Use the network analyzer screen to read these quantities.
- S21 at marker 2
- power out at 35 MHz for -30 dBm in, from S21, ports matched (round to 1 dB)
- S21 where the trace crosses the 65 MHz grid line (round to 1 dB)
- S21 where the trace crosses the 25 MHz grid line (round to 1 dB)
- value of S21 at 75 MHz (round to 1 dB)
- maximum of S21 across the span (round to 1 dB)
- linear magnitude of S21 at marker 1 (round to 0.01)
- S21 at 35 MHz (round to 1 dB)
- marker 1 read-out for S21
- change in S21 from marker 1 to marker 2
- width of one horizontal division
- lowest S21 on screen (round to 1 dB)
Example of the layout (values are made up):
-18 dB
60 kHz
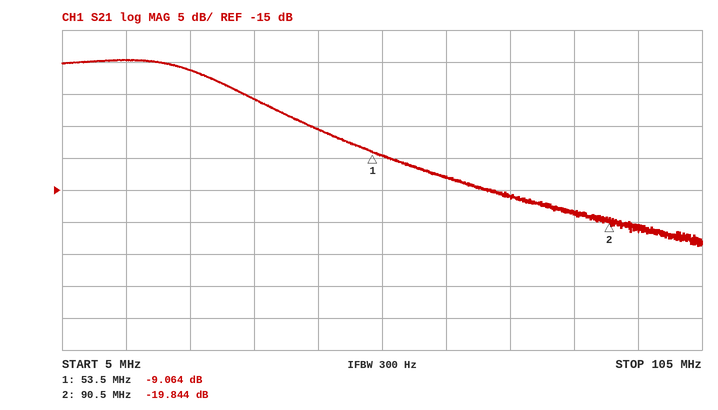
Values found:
-19.844 dB
-31 dBm
-13 dB
4 dB
-16 dB
5 dB
0.35
-1 dB
-9.064 dB
-10.780 dB
10 MHz
-24 dB
